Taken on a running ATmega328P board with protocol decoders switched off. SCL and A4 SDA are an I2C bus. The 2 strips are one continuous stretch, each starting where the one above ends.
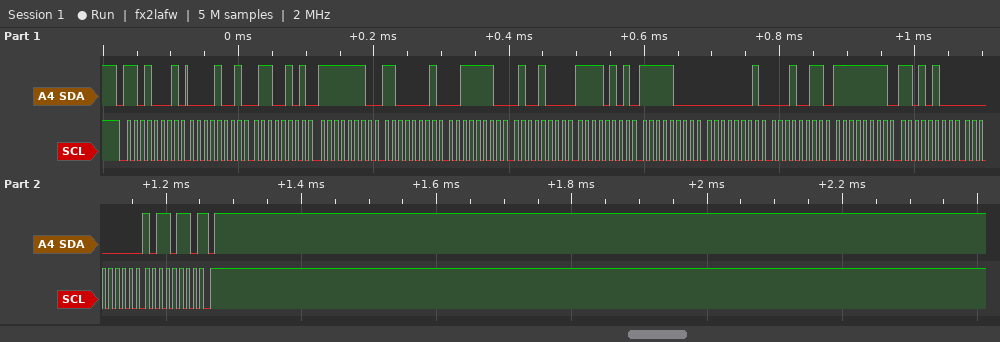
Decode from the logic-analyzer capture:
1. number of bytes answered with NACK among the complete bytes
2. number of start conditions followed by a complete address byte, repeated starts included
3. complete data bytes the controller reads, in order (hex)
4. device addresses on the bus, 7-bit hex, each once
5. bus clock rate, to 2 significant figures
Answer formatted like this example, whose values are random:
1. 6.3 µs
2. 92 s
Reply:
1. 1
2. 1
3. 09 65 FE C1 3E 48 F5 F8 01 13 FF D4 00 B6
4. 0x68
5. 100 kHz
